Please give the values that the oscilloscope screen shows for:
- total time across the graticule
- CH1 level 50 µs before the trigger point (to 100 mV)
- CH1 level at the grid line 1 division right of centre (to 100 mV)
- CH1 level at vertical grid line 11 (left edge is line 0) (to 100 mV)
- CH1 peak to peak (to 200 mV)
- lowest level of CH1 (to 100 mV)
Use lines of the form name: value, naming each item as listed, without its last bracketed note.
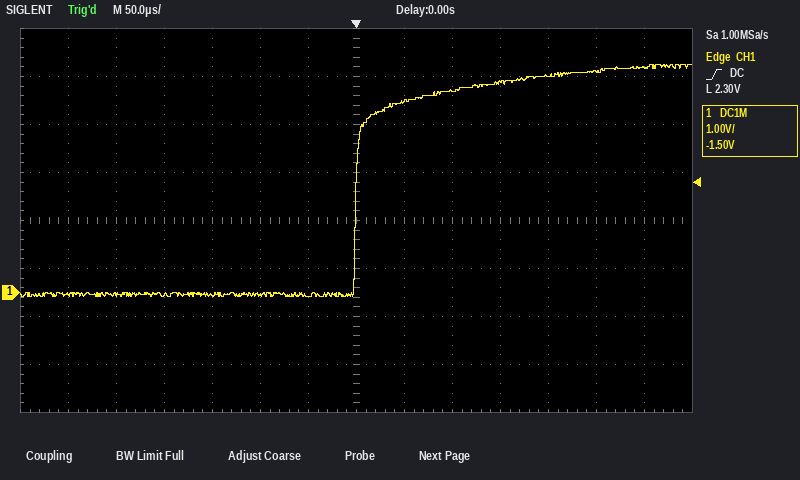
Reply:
total time across the graticule: 700 µs
CH1 level 50 µs before the trigger point: -100 mV
CH1 level at the grid line 1 division right of centre: 4.0 V
CH1 level at vertical grid line 11 (left edge is line 0): 4.5 V
CH1 peak to peak: 4.8 V
lowest level of CH1: -100 mV
